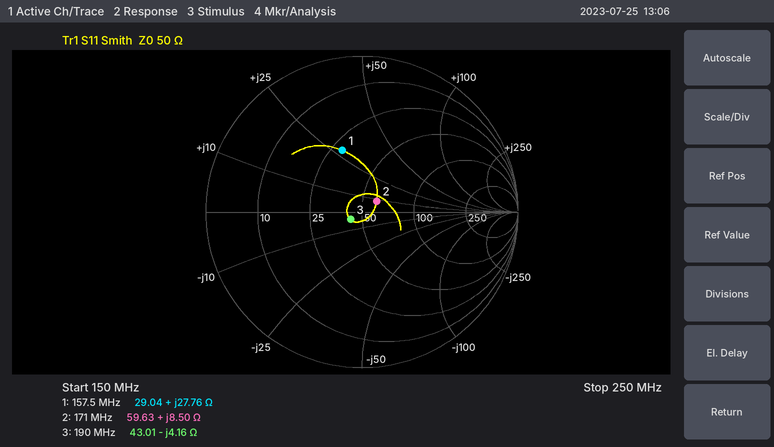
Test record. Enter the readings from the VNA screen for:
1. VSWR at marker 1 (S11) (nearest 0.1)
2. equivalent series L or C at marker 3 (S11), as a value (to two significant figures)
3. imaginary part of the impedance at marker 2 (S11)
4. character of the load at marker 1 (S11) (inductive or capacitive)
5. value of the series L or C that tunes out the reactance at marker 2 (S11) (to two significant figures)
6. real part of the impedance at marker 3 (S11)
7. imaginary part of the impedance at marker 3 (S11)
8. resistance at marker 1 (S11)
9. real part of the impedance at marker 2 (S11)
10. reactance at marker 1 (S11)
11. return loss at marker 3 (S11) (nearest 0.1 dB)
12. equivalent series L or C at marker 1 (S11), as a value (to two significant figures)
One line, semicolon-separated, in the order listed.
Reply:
2.4; 200 pF; +8.50 Ω; inductive; 110 pF; 43.01 Ω; -4.16 Ω; 29.04 Ω; 59.63 Ω; +27.76 Ω; 21.2 dB; 28 nH
